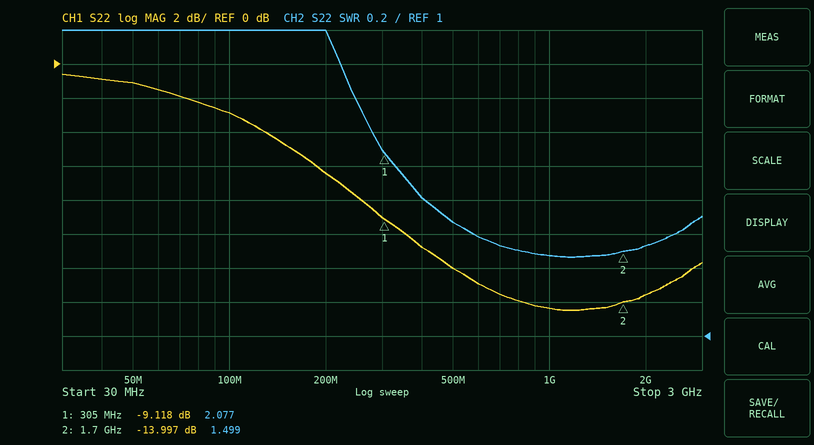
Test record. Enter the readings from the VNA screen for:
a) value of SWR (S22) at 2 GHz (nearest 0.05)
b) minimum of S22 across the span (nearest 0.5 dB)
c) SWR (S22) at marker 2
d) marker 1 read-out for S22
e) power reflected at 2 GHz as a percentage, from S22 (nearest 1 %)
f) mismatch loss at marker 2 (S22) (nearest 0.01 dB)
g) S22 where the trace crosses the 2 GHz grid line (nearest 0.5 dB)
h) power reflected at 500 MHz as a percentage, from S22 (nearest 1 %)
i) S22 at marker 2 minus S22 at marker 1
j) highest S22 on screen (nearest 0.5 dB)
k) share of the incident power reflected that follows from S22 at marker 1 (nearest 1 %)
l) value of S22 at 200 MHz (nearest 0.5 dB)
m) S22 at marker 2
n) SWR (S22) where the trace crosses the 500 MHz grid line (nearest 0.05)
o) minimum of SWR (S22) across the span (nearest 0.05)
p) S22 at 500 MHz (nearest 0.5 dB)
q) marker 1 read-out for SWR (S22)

1.55
-14.5 dB
1.499
-9.118 dB
4 %
0.18 dB
-13.5 dB
6 %
-4.879 dB
-0.5 dB
12 %
-6.5 dB
-13.997 dB
1.65
1.45
-12.0 dB
2.077
